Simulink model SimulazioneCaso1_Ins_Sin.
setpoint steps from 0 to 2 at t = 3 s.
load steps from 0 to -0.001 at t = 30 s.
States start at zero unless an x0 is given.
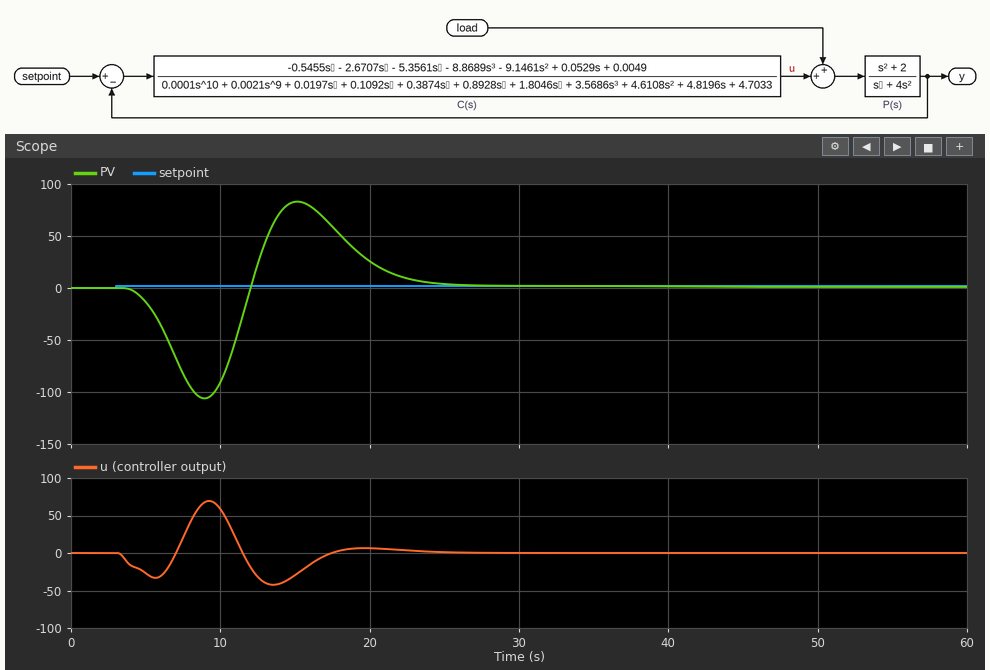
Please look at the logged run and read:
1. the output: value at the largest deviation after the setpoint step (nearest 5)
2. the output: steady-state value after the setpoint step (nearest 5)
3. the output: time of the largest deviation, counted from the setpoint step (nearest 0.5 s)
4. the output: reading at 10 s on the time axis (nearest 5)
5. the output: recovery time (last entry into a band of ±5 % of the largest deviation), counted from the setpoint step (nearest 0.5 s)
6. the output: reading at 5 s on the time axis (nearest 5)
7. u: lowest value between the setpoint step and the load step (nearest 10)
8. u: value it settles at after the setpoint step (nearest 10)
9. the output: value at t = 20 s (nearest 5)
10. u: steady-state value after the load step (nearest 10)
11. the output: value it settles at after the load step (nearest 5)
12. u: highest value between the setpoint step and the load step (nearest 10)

-105
0
6.0 s
-90
20.0 s
-15
-40
0
25
0
0
70
